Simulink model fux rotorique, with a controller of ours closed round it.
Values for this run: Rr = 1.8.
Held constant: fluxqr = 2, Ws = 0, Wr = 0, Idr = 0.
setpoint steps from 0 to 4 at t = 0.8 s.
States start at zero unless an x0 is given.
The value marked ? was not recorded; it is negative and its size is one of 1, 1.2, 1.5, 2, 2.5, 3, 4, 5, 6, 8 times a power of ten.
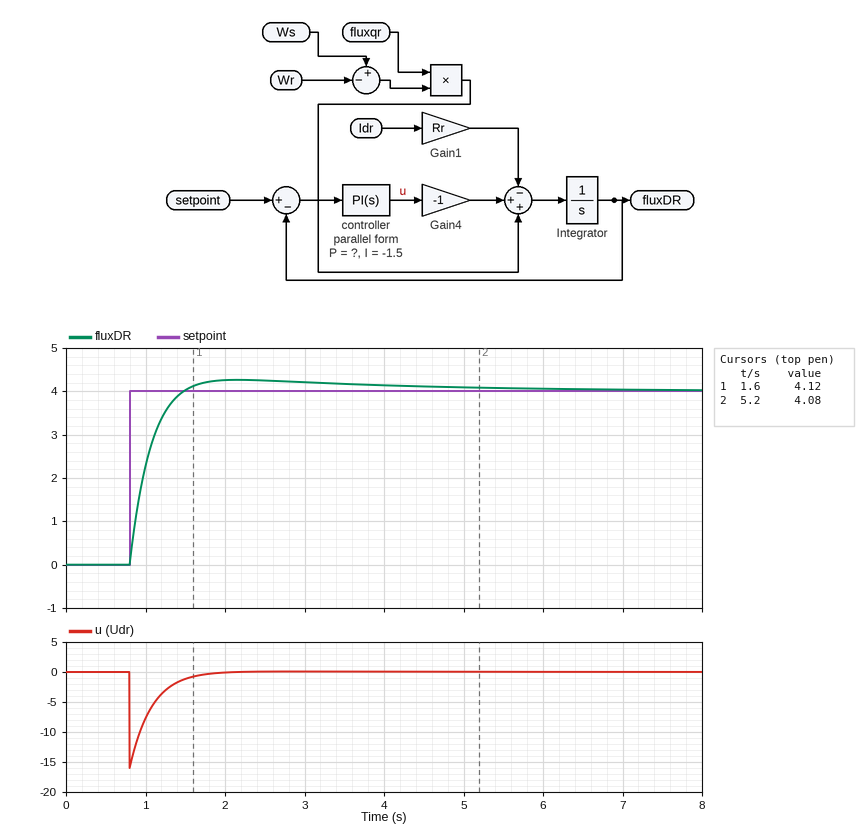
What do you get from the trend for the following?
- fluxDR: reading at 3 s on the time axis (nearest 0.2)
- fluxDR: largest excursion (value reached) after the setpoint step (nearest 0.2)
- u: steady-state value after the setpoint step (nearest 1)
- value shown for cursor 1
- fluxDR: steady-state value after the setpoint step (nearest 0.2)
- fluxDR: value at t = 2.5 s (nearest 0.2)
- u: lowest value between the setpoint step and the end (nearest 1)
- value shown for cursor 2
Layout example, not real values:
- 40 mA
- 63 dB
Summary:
- 4.2
- 4.2
- 0
- 4.12
- 4.0
- 4.2
- -16
- 4.08
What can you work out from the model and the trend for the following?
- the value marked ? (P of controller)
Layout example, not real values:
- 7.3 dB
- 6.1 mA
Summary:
- -4
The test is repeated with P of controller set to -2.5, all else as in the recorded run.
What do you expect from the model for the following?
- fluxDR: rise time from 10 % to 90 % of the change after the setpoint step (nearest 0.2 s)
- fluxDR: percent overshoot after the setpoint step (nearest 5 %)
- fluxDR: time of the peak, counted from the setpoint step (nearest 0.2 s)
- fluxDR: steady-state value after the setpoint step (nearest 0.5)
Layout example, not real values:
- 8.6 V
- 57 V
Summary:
- 0.6 s
- 15 %
- 1.6 s
- 4.0
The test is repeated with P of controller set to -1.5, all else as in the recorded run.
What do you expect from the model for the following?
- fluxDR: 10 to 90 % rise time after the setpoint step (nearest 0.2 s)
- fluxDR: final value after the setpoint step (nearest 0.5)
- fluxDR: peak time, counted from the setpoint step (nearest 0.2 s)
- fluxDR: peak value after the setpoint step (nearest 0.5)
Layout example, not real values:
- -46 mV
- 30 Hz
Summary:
- 0.8 s
- 4.0
- 1.8 s
- 5.0
